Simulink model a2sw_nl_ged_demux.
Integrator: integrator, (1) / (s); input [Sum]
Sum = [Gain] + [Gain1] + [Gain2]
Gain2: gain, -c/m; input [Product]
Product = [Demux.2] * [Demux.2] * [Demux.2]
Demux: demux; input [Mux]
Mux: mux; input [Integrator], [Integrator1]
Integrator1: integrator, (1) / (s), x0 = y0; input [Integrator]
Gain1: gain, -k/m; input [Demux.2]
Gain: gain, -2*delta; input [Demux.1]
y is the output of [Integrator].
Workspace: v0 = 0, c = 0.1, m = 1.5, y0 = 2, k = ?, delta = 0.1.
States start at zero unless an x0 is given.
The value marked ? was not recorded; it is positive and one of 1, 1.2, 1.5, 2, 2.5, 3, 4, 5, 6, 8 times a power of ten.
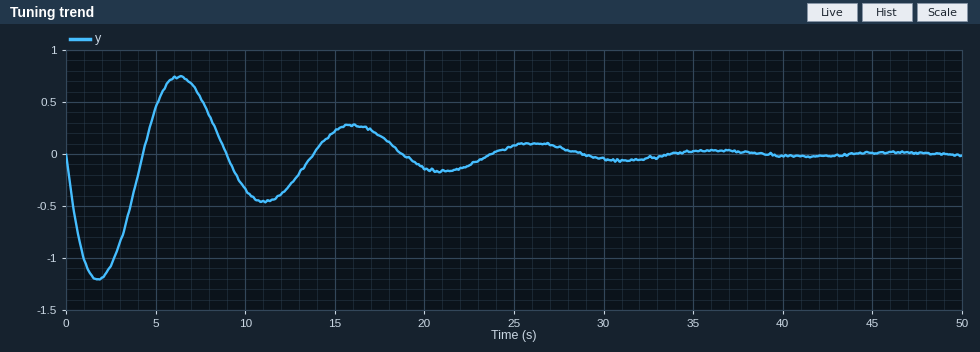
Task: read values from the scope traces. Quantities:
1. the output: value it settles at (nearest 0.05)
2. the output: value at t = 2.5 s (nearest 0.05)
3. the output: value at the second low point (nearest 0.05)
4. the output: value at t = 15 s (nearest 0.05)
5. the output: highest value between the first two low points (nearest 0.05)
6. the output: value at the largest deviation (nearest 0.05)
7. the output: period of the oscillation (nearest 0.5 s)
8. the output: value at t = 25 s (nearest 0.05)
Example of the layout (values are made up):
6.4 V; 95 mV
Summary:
0.00; -1.05; -0.45; 0.20; 0.75; -1.20; 9.5 s; 0.10
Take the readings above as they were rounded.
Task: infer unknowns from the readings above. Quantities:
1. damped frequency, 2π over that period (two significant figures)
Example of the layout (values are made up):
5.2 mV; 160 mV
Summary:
0.66 rad/s
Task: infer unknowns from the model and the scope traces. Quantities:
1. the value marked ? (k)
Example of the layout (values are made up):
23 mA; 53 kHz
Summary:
0.6
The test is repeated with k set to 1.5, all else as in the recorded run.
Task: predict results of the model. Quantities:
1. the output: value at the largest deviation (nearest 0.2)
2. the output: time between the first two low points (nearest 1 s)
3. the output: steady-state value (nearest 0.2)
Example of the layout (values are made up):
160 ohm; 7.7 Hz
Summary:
-1.8; 6 s; 0.0
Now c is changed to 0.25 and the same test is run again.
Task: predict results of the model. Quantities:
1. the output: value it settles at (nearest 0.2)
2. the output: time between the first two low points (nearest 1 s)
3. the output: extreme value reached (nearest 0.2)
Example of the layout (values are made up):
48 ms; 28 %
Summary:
0.0; 8 s; -1.4
